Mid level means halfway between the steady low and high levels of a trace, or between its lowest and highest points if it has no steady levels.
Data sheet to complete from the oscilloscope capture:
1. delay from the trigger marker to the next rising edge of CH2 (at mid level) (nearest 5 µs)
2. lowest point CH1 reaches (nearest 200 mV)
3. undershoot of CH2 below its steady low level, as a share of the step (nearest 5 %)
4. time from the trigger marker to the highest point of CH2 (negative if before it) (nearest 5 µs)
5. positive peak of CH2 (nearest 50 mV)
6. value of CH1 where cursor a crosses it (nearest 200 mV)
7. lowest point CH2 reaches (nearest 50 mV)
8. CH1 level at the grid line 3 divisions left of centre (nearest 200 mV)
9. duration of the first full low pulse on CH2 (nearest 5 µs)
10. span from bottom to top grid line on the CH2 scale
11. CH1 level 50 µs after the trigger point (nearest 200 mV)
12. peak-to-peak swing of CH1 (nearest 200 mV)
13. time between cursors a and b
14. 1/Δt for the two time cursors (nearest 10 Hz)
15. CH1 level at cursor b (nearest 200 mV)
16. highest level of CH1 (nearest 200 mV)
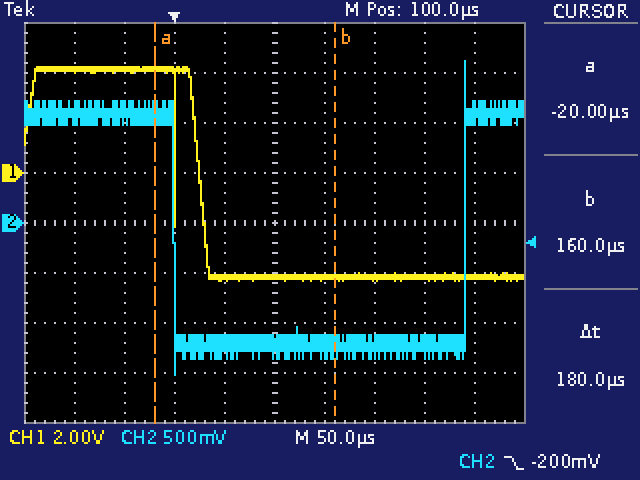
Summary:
290 µs
-4.4 V
15 %
+290 µs
1.60 V
4.2 V
-1.50 V
4.2 V
290 µs
4 V
-4.2 V
8.6 V
180 µs
5.56 kHz
-4.2 V
4.2 V
